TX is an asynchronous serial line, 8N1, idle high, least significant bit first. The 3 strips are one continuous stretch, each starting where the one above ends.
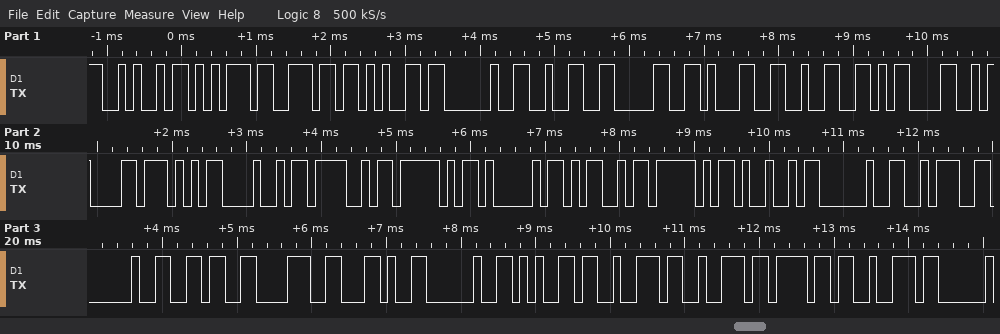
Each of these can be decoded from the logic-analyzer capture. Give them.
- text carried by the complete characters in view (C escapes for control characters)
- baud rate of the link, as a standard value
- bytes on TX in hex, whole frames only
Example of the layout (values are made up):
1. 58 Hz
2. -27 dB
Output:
1. "June 2012\r\nWHO_AM_I : 68, error"
2. 9600 baud
3. 0x4A 0x75 0x6E 0x65 0x20 0x32 0x30 0x31 0x32 0x0D 0x0A 0x57 0x48 0x4F 0x5F 0x41 0x4D 0x5F 0x49 0x20 0x3A 0x20 0x36 0x38 0x2C 0x20 0x65 0x72 0x72 0x6F 0x72
